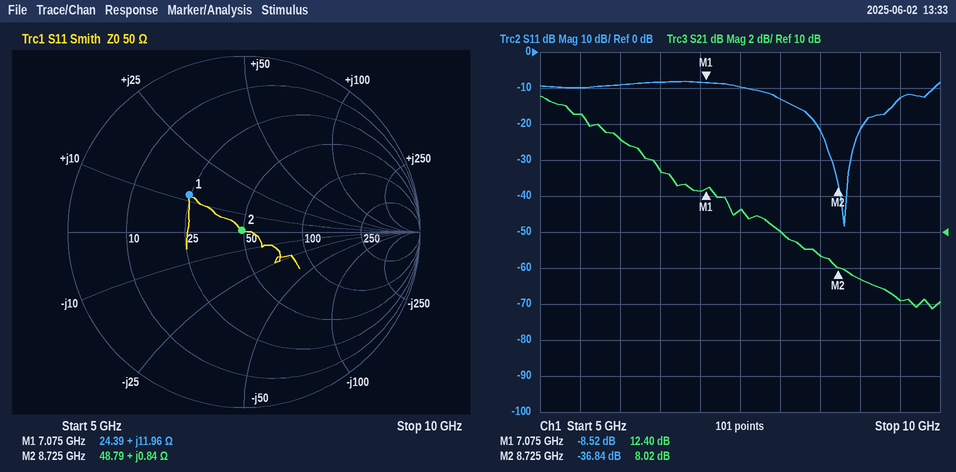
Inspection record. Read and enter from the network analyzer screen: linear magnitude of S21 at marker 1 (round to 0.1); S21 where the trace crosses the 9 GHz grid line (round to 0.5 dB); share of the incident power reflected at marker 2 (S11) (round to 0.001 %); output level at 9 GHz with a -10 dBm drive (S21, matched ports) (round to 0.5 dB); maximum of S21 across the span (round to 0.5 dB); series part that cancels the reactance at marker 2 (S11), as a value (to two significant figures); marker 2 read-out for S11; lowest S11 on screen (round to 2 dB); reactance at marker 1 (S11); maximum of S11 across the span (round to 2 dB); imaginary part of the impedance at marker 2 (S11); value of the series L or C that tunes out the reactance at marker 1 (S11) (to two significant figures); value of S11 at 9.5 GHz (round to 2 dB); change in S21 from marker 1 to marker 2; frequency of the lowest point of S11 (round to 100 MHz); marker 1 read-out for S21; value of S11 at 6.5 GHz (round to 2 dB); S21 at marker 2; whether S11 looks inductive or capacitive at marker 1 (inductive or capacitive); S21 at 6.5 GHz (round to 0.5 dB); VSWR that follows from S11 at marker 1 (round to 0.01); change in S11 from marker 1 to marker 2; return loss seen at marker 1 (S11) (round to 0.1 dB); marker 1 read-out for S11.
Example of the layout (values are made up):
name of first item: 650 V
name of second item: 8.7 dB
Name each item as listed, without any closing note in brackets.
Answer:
linear magnitude of S21 at marker 1: 4.2
S21 where the trace crosses the 9 GHz grid line: 7.5 dB
share of the incident power reflected at marker 2 (S11): 0.021 %
output level at 9 GHz with a -10 dBm drive (S21, matched ports): -2.5 dBm
maximum of S21 across the span: 17.5 dB
series part that cancels the reactance at marker 2 (S11), as a value: 22 pF
marker 2 read-out for S11: -36.84 dB
lowest S11 on screen: -48 dB
reactance at marker 1: +11.96 Ω
maximum of S11 across the span: -8 dB
imaginary part of the impedance at marker 2: +0.84 Ω
value of the series L or C that tunes out the reactance at marker 1 (S11): 1.9 pF
value of S11 at 9.5 GHz: -12 dB
change in S21 from marker 1 to marker 2: -4.38 dB
frequency of the lowest point of S11: 8.8 GHz
marker 1 read-out for S21: 12.40 dB
value of S11 at 6.5 GHz: -8 dB
S21 at marker 2: 8.02 dB
whether S11 looks inductive or capacitive at marker 1: inductive
S21 at 6.5 GHz: 13.5 dB
VSWR that follows from S11 at marker 1: 2.20
change in S11 from marker 1 to marker 2: -28.32 dB
return loss seen at marker 1 (S11): 8.5 dB
marker 1 read-out for S11: -8.52 dB
